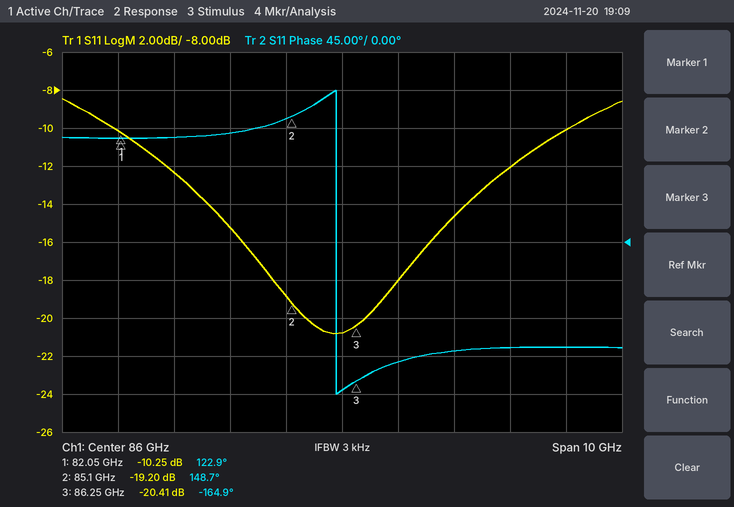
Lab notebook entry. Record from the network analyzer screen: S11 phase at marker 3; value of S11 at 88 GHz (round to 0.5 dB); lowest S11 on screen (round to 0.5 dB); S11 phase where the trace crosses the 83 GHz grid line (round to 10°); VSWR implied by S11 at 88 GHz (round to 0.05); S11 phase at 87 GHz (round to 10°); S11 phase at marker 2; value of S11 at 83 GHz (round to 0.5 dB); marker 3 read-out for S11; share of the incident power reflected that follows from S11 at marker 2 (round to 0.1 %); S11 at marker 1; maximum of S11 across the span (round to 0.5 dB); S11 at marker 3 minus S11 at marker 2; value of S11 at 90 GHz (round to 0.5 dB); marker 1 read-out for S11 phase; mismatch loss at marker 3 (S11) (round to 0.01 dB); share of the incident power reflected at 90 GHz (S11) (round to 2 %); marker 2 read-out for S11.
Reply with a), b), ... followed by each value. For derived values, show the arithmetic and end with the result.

a) -164.9°
b) -14.5 dB
c) -21.0 dB
d) 120°
e) |Γ| = 10^(-14.5/20) = 0.1884; VSWR = (1 + 0.1884)/(1 − 0.1884) ≈ 1.46, so 1.45 to the nearest 0.05
f) -140°
g) 148.7°
h) -12.5 dB
i) -20.41 dB
j) 10^(-19.2/10) ≈ 1.2 %
k) -10.25 dB
l) -8.5 dB
m) -20.41 − (-19.2) = -1.21 dB
n) -10.0 dB
o) 122.9°
p) −10 log10(1 − 10^(-20.41/10)) ≈ 0.04 dB
q) 10^(-10/10) ≈ 10 %
r) -19.20 dB
